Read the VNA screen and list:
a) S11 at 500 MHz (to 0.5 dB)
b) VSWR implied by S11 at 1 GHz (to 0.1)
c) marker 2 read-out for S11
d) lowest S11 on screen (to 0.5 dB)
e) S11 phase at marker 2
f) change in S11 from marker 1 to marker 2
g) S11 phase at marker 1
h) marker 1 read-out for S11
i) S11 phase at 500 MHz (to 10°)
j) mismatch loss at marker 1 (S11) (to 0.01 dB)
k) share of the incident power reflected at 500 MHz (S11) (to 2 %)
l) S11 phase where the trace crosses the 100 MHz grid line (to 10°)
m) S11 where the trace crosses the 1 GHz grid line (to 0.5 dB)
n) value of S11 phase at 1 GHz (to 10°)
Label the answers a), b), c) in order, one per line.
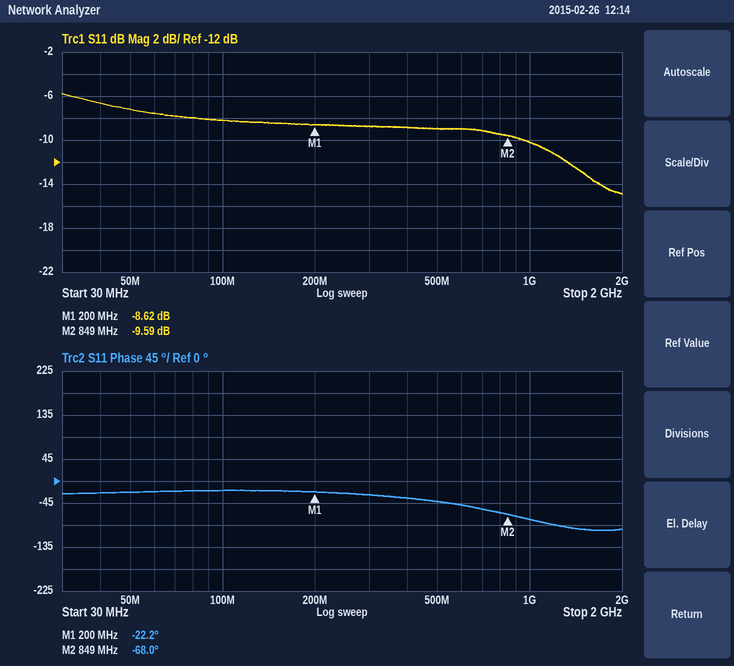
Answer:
a) -9.0 dB
b) 1.9
c) -9.59 dB
d) -15.0 dB
e) -68.0°
f) -0.97 dB
g) -22.2°
h) -8.62 dB
i) -40°
j) 0.64 dB
k) 12 %
l) -20°
m) -10.0 dB
n) -80°
